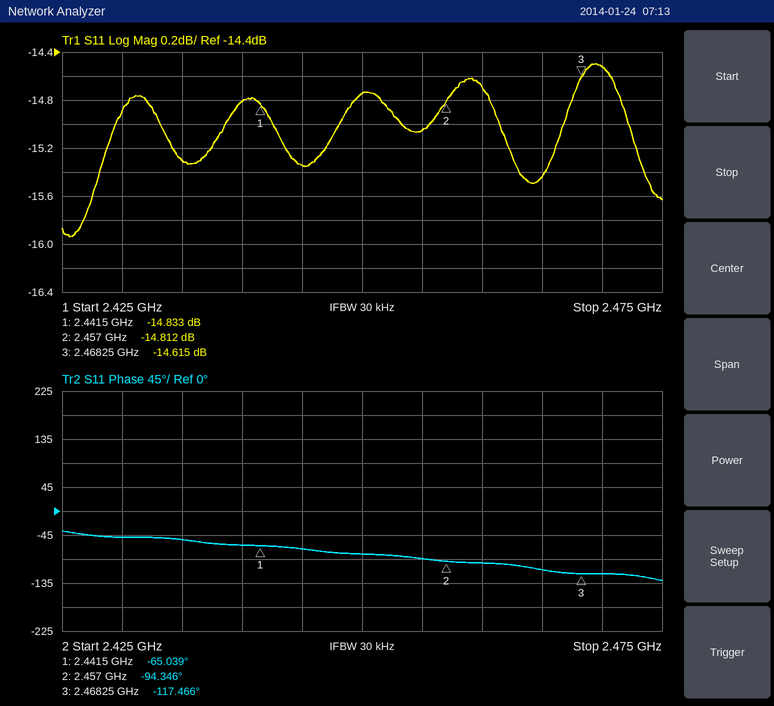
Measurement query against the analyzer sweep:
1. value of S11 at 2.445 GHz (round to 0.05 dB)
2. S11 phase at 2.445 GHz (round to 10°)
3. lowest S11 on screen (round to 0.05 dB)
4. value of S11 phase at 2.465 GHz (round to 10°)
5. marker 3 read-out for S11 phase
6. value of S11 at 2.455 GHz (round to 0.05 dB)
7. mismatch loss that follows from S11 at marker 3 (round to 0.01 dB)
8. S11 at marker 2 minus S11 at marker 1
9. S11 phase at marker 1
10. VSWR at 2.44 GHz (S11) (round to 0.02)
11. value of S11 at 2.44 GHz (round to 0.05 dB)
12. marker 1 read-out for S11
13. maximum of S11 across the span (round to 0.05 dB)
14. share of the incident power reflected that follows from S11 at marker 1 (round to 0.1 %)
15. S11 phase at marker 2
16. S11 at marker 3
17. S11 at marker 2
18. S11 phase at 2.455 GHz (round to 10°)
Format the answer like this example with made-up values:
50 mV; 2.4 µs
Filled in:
-15.35 dB; -70°; -15.95 dB; -110°; -117.466°; -15.05 dB; 0.15 dB; 0.021 dB; -65.039°; 1.44; -14.80 dB; -14.833 dB; -14.50 dB; 3.3 %; -94.346°; -14.615 dB; -14.812 dB; -90°
